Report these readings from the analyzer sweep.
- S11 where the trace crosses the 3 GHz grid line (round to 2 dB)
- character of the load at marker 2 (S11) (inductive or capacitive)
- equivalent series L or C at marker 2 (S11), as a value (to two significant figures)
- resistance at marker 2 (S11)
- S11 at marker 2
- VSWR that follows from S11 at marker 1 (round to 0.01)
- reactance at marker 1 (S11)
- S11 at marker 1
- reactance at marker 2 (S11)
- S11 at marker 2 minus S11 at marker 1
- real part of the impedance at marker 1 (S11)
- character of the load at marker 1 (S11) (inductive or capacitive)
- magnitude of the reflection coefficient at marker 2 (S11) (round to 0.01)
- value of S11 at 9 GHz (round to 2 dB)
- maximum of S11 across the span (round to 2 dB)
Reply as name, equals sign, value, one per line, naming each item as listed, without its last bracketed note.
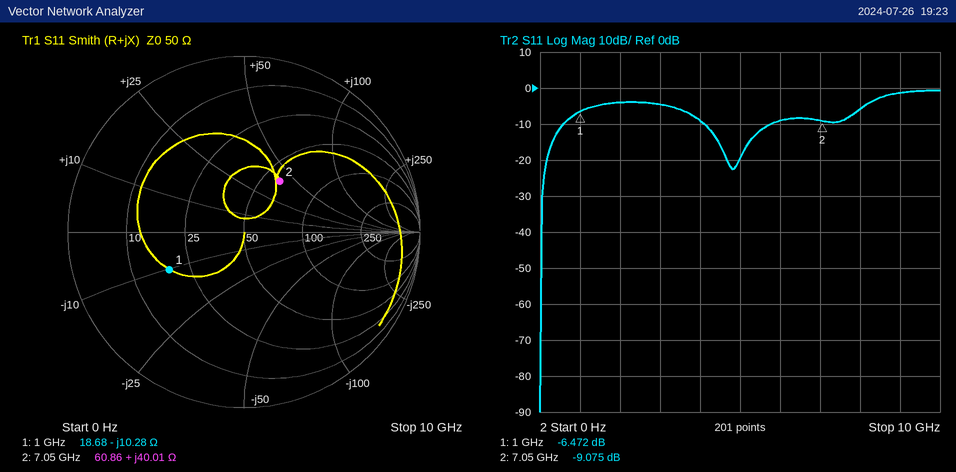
S11 where the trace crosses the 3 GHz grid line = -4 dB
character of the load at marker 2 (S11) = inductive
equivalent series L or C at marker 2 (S11), as a value = 900 pH
resistance at marker 2 = 60.86 Ω
S11 at marker 2 = -9.075 dB
VSWR that follows from S11 at marker 1 = 2.81
reactance at marker 1 = -10.28 Ω
S11 at marker 1 = -6.472 dB
reactance at marker 2 = +40.01 Ω
S11 at marker 2 minus S11 at marker 1 = -2.603 dB
real part of the impedance at marker 1 = 18.68 Ω
character of the load at marker 1 (S11) = capacitive
magnitude of the reflection coefficient at marker 2 (S11) = 0.35
value of S11 at 9 GHz = -2 dB
maximum of S11 across the span = 0 dB
